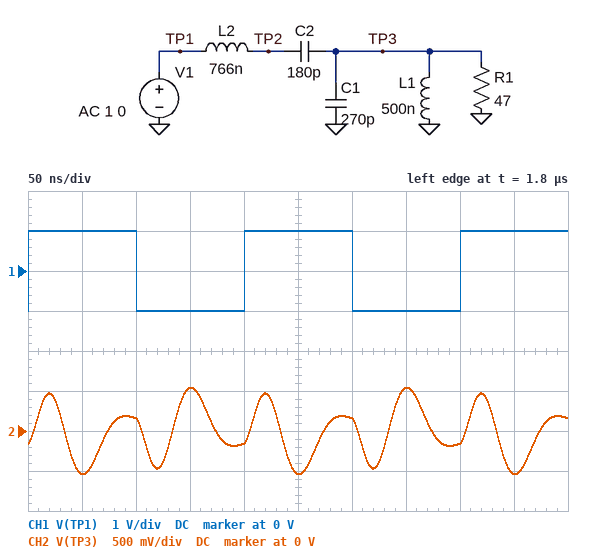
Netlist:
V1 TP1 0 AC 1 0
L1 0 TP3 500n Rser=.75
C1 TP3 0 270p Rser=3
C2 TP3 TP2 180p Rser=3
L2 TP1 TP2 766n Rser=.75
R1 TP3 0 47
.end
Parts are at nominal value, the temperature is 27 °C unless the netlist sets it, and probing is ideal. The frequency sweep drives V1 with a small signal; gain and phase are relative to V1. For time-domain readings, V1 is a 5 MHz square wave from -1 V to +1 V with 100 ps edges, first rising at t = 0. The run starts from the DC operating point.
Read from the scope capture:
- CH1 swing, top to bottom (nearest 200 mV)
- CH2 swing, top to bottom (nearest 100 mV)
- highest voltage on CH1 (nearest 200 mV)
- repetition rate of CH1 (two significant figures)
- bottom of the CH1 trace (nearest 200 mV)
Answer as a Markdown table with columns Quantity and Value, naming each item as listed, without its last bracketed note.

| Quantity | Value |
|---|---|
| CH1 swing, top to bottom | 2.0 V |
| CH2 swing, top to bottom | 1.1 V |
| highest voltage on CH1 | 1.0 V |
| repetition rate of CH1 | 5.0 MHz |
| bottom of the CH1 trace | -1.0 V |
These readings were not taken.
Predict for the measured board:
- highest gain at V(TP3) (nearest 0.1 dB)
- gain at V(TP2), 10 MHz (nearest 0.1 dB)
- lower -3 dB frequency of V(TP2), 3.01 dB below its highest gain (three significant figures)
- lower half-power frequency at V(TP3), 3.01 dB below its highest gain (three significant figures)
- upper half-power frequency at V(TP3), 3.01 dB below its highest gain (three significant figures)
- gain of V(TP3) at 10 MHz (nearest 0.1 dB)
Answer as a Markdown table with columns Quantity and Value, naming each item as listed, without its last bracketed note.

| Quantity | Value |
|---|---|
| highest gain at V(TP3) | -0.4 dB |
| gain at V(TP2), 10 MHz | 5.6 dB |
| lower -3 dB frequency of V(TP2), 3.01 dB below its highest gain | 6.50 MHz |
| lower half-power frequency at V(TP3), 3.01 dB below its highest gain | 8.68 MHz |
| upper half-power frequency at V(TP3), 3.01 dB below its highest gain | 20.6 MHz |
| gain of V(TP3) at 10 MHz | -0.8 dB |
